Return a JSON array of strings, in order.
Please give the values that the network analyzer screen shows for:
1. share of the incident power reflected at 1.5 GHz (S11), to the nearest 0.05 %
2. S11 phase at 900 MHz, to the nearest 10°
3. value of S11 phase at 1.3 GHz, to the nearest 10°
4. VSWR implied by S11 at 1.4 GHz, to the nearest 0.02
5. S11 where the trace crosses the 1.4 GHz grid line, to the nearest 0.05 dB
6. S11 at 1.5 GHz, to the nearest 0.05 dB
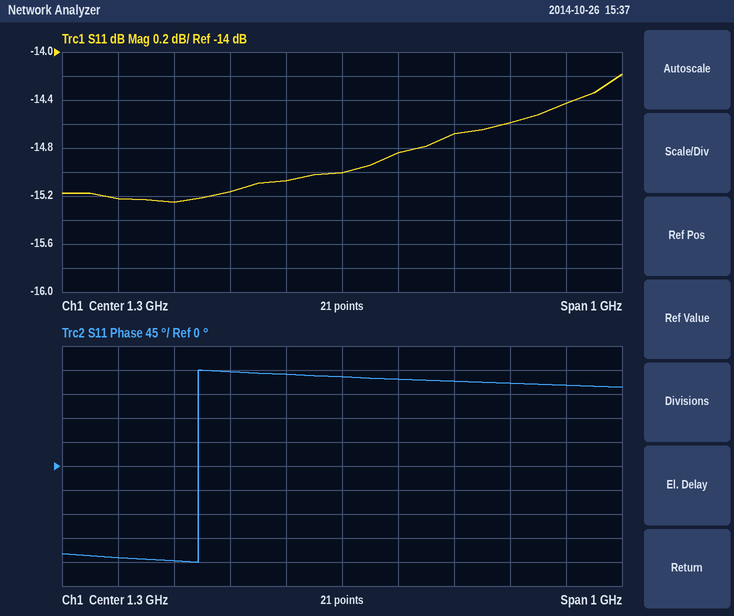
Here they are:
["3.40 %", "-170°", "170°", "1.44", "-14.85 dB", "-14.70 dB"]
